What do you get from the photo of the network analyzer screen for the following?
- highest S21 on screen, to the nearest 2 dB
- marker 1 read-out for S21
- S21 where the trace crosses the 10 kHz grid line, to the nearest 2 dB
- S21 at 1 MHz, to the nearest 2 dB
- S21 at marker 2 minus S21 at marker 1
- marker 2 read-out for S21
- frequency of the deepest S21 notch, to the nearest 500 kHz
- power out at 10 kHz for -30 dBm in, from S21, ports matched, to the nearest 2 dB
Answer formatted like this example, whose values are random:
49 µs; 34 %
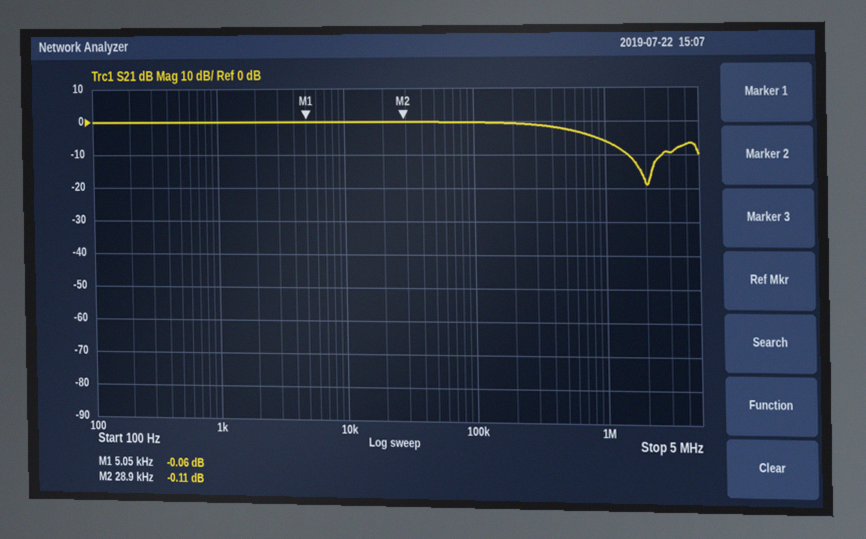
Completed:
0 dB; -0.06 dB; 0 dB; -6 dB; -0.05 dB; -0.11 dB; 2.0 MHz; -30 dBm
